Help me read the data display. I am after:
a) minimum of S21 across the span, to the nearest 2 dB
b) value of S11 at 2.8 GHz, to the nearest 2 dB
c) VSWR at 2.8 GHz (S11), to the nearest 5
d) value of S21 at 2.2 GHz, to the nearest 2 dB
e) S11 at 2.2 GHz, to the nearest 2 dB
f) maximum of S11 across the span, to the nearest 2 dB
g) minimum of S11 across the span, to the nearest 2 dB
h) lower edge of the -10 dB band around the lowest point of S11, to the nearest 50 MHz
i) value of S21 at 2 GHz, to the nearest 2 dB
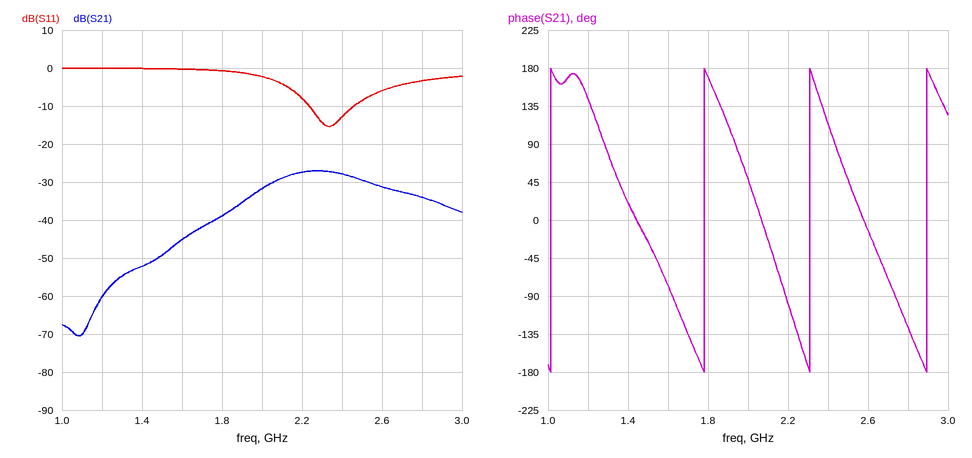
-70 dB
-4 dB
5
-28 dB
-8 dB
0 dB
-16 dB
2.25 GHz
-32 dB
